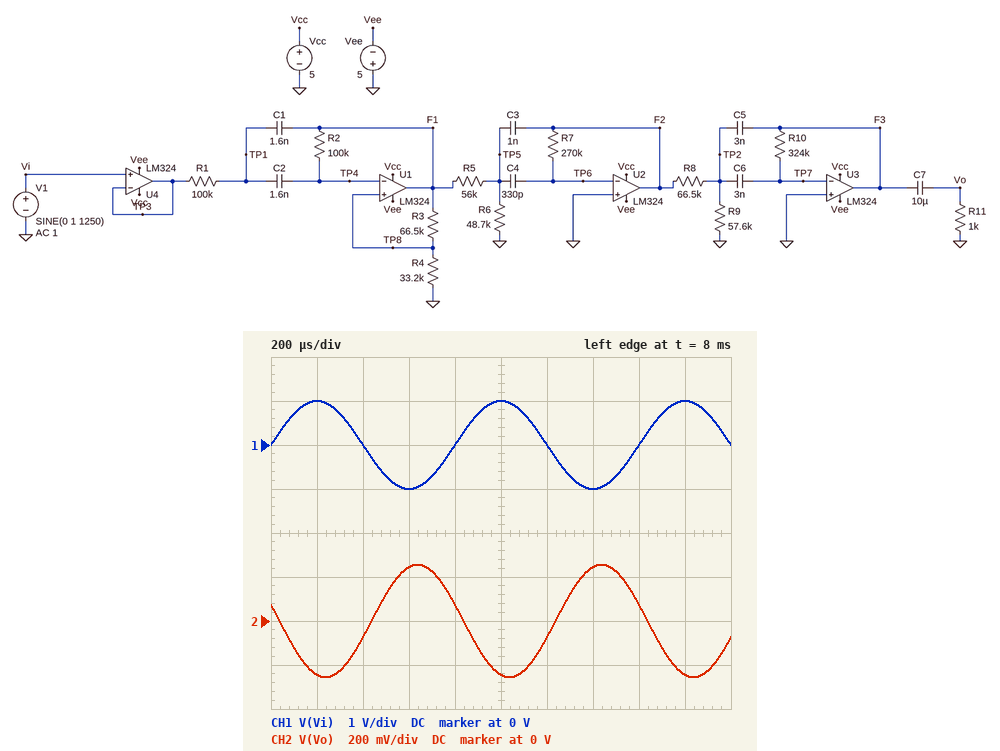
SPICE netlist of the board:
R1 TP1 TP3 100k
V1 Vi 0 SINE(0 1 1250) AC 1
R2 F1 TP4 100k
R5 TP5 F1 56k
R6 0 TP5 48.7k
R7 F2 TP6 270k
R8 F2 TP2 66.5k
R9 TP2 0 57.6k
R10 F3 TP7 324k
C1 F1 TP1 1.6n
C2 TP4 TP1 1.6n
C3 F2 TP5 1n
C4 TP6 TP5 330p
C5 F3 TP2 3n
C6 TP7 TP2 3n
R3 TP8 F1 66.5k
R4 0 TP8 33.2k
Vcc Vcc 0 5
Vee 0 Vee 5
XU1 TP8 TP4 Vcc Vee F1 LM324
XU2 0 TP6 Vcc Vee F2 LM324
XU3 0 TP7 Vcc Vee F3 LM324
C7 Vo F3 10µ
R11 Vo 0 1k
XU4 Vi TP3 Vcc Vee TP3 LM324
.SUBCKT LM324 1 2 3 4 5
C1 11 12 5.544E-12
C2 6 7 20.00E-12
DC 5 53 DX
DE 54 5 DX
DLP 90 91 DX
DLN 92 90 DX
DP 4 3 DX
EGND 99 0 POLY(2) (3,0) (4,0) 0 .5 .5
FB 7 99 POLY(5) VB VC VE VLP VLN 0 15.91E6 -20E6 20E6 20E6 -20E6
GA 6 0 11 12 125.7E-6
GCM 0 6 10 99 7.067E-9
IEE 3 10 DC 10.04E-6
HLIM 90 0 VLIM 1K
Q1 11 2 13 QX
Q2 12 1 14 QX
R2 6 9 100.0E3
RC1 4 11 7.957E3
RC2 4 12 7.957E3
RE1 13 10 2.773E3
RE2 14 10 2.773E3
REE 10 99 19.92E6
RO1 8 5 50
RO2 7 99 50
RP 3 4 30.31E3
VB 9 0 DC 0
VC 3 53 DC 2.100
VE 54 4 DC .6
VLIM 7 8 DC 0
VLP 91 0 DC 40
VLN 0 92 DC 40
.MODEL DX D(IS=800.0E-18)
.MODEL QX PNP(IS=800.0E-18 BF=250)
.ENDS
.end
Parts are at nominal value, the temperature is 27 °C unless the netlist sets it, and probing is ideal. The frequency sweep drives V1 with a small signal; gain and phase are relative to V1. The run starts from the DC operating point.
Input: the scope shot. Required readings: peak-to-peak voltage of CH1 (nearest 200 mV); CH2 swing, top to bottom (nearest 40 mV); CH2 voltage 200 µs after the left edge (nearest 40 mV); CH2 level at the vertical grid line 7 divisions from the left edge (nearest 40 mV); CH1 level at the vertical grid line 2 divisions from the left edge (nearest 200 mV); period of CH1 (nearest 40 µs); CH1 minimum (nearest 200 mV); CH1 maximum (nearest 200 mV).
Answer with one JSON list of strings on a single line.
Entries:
["2.0 V", "520 mV", "-240 mV", "240 mV", "0 V", "800 µs", "-1.0 V", "1.0 V"]
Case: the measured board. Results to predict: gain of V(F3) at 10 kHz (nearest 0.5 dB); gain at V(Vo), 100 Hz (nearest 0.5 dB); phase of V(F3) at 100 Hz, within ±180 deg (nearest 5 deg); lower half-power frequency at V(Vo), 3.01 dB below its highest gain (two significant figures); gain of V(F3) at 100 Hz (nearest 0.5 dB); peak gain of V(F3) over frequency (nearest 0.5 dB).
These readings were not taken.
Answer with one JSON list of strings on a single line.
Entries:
["-49.0 dB", "-59.0 dB", "75 deg", "490 Hz", "-59.0 dB", "-10.5 dB"]
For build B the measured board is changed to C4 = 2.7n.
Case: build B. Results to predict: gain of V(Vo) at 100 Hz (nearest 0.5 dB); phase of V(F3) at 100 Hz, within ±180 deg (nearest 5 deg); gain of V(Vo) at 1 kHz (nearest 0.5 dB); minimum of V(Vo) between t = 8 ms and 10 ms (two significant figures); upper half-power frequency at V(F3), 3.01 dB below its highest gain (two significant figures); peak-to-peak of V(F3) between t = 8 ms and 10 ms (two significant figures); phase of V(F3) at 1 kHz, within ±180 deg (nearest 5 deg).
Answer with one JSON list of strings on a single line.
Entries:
["-40.5 dB", "70 deg", "10.5 dB", "-2.4 V", "1.3 kHz", "4.8 V", "135 deg"]
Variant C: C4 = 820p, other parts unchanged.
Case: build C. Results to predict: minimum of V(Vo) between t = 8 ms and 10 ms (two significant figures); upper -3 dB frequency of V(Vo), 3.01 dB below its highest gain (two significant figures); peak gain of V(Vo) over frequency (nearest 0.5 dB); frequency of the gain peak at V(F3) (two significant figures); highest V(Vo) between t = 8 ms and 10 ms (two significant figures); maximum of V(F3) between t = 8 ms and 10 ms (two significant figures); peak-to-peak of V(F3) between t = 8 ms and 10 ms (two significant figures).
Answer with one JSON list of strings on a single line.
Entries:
["-770 mV", "2.1 kHz", "-2.0 dB", "730 Hz", "770 mV", "760 mV", "1.5 V"]
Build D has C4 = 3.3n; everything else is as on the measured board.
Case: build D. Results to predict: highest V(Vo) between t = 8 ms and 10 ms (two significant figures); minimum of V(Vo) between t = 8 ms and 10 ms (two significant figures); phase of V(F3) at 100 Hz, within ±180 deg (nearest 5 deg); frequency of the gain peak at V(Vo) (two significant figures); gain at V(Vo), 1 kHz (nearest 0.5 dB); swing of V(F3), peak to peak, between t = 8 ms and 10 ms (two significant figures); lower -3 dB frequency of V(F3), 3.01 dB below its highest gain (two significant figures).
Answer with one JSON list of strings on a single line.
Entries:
["2.3 V", "-2.3 V", "70 deg", "810 Hz", "11.5 dB", "4.7 V", "520 Hz"]
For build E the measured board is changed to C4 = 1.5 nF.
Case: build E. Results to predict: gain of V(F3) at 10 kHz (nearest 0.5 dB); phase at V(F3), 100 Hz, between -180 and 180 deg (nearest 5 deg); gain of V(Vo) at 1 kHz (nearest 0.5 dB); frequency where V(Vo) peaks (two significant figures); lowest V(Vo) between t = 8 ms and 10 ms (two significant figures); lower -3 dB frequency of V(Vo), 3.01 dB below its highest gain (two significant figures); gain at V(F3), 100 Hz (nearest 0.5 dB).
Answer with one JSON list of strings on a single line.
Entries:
["-49.5 dB", "70 deg", "4.5 dB", "1.2 kHz", "-1.7 V", "520 Hz", "-45.5 dB"]
